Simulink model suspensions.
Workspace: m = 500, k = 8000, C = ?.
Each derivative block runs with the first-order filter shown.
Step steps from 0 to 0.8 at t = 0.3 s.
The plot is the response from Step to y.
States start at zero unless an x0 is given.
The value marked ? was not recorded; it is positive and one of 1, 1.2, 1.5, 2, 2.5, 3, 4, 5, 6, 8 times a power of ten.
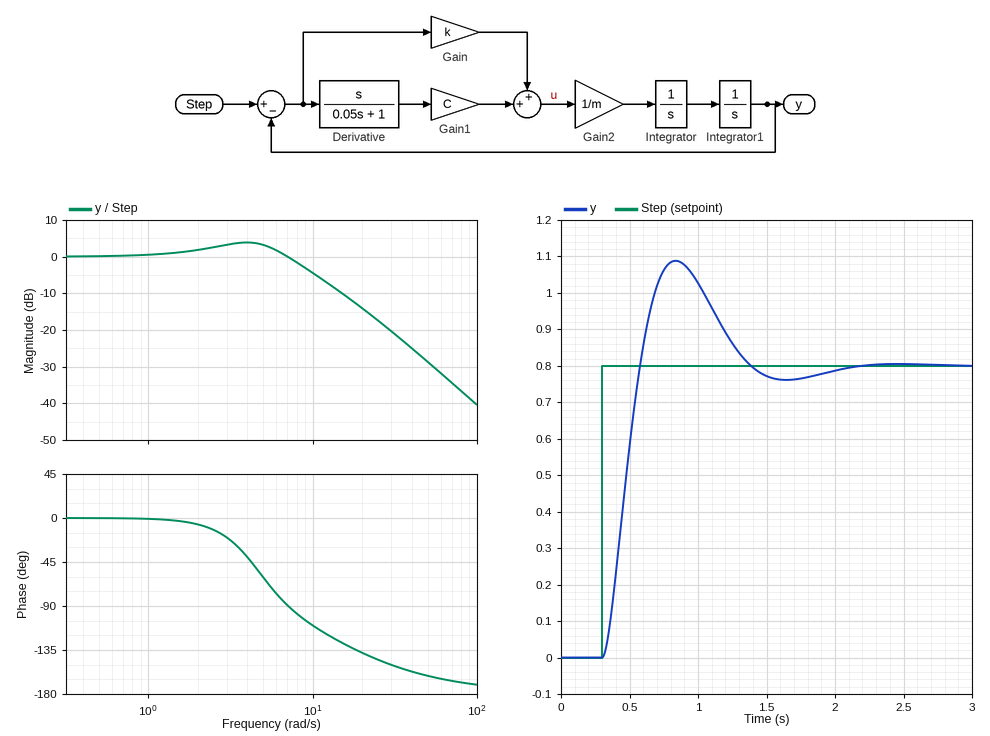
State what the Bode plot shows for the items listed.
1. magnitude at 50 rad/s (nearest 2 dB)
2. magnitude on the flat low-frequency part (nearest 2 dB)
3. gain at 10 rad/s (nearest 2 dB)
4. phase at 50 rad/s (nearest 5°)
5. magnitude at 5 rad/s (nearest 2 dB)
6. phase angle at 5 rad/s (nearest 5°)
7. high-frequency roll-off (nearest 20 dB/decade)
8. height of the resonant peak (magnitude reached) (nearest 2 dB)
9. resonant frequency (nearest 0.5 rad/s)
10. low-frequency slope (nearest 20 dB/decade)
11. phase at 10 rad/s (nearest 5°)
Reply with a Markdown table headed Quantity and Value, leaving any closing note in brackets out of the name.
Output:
| Quantity | Value |
|---|---|
| magnitude at 50 rad/s | -28 dB |
| magnitude on the flat low-frequency part | 0 dB |
| gain at 10 rad/s | -4 dB |
| phase at 50 rad/s | -160° |
| magnitude at 5 rad/s | 4 dB |
| phase angle at 5 rad/s | -60° |
| high-frequency roll-off | -40 dB/decade |
| height of the resonant peak (magnitude reached) | 4 dB |
| resonant frequency | 4.0 rad/s |
| low-frequency slope | 0 dB/decade |
| phase at 10 rad/s | -110° |
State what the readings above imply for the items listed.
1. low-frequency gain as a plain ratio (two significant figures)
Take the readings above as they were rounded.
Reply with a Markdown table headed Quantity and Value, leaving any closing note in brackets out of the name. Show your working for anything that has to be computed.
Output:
| Quantity | Value |
|---|---|
| low-frequency gain as a plain ratio | 10^(0 / 20) = 1.0 |
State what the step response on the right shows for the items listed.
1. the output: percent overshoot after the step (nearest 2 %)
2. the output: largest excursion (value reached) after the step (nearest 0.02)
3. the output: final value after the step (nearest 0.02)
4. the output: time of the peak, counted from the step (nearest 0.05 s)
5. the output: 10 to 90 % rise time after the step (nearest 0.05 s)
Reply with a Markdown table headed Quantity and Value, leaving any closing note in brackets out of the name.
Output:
| Quantity | Value |
|---|---|
| the output: percent overshoot after the step | 36 % |
| the output: largest excursion (value reached) after the step | 1.08 |
| the output: final value after the step | 0.80 |
| the output: time of the peak, counted from the step | 0.55 s |
| the output: 10 to 90 % rise time after the step | 0.20 s |
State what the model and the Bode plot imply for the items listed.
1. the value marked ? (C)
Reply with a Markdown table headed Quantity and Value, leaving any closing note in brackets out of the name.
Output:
| Quantity | Value |
|---|---|
| the value marked ? | 2000 |
